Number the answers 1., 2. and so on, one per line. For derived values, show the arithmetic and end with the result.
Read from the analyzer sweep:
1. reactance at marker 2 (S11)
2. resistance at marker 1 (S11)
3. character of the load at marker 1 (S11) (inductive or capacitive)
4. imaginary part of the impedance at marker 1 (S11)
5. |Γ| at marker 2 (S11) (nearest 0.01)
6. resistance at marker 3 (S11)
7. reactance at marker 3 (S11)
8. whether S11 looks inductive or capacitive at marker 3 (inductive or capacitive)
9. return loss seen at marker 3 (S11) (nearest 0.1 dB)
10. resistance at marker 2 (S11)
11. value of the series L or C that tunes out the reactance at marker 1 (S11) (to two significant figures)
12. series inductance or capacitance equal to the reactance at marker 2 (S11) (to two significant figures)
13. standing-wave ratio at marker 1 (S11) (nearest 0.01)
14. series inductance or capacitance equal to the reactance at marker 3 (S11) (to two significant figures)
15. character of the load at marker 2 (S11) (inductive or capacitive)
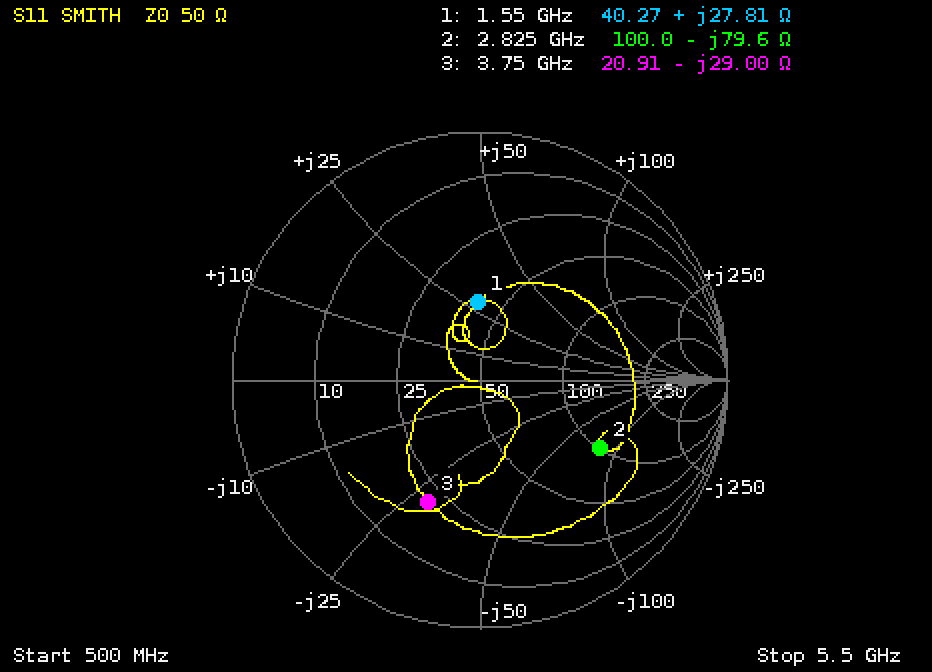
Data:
1. -79.6 Ω
2. 40.27 Ω
3. inductive
4. +27.81 Ω
5. 0.55
6. 20.91 Ω
7. -29.00 Ω
8. capacitive
9. 5.4 dB
10. 100.0 Ω
11. C = 1/(2π × 1.55 GHz × 27.81 Ω) ≈ 3.7 pF
12. C = 1/(2π × 2.825 GHz × 79.6 Ω) ≈ 708 fF, so 710 fF to two significant figures
13. 1.91
14. C = 1/(2π × 3.75 GHz × 29 Ω) ≈ 1.5 pF
15. capacitive
